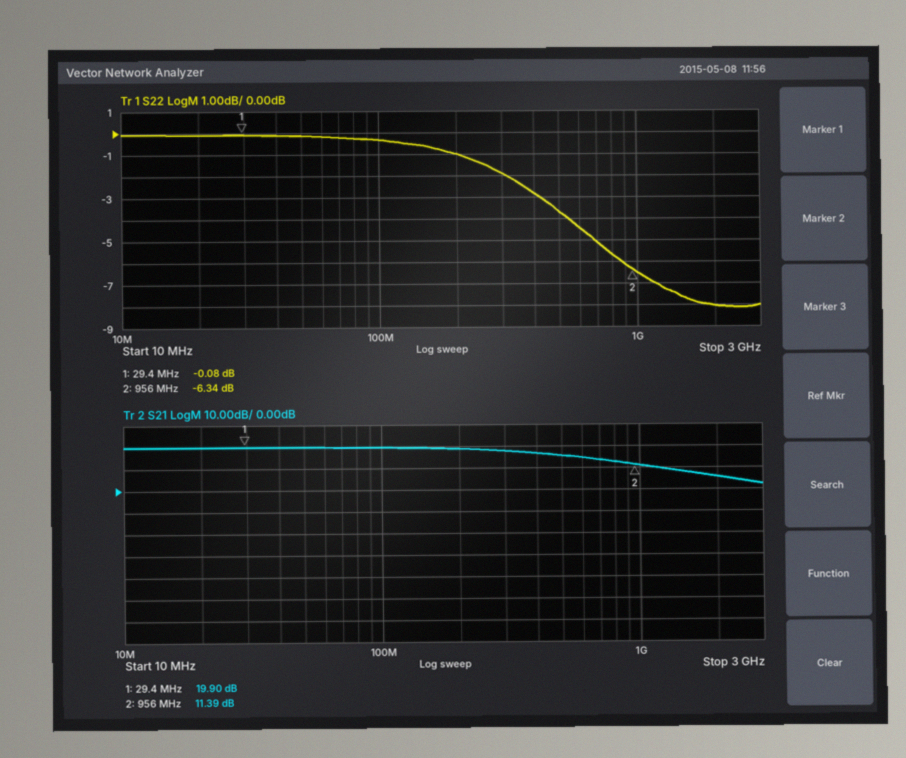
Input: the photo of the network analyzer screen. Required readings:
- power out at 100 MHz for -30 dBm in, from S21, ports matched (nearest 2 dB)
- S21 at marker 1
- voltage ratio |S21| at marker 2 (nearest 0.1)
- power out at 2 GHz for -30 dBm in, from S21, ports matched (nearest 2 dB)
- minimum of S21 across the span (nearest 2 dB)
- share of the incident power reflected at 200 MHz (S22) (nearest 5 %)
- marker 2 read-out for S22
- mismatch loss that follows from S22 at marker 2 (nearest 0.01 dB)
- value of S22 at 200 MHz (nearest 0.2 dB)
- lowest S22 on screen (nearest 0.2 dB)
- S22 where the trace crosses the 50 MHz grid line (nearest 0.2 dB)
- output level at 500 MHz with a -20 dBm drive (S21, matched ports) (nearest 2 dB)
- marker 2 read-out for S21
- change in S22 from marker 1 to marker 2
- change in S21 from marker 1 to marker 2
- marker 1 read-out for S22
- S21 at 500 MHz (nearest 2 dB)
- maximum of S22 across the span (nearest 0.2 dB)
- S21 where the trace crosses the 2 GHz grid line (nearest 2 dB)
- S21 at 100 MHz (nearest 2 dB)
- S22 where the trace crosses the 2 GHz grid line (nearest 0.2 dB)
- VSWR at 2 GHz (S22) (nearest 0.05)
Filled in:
-10 dBm
19.90 dB
3.7
-24 dBm
2 dB
80 %
-6.34 dB
1.15 dB
-1.0 dB
-8.2 dB
-0.2 dB
-4 dBm
11.39 dB
-6.26 dB
-8.51 dB
-0.08 dB
16 dB
0.0 dB
6 dB
20 dB
-8.0 dB
2.30
